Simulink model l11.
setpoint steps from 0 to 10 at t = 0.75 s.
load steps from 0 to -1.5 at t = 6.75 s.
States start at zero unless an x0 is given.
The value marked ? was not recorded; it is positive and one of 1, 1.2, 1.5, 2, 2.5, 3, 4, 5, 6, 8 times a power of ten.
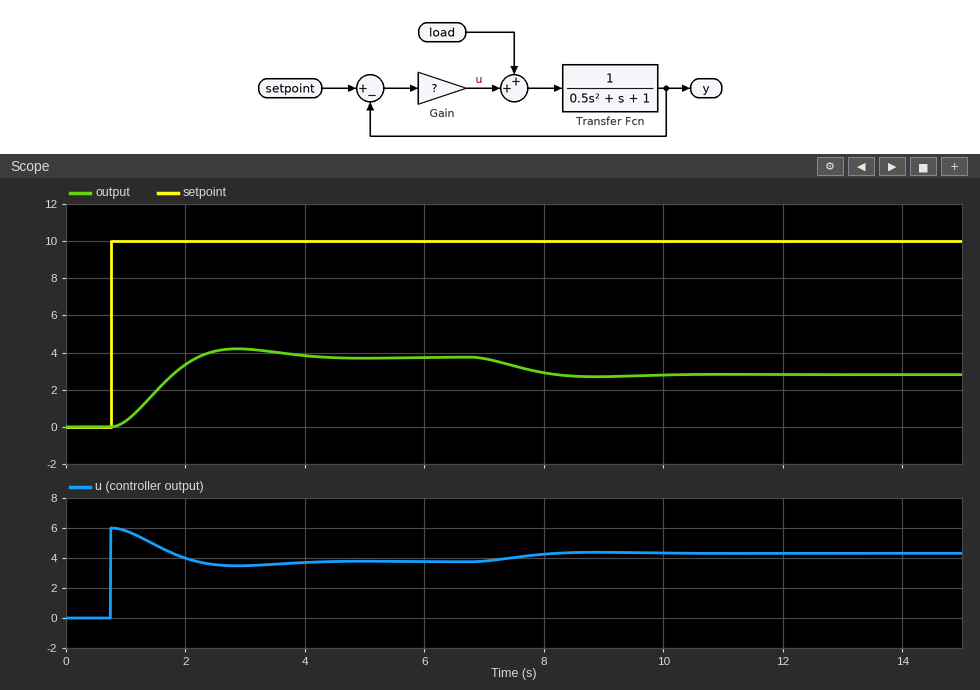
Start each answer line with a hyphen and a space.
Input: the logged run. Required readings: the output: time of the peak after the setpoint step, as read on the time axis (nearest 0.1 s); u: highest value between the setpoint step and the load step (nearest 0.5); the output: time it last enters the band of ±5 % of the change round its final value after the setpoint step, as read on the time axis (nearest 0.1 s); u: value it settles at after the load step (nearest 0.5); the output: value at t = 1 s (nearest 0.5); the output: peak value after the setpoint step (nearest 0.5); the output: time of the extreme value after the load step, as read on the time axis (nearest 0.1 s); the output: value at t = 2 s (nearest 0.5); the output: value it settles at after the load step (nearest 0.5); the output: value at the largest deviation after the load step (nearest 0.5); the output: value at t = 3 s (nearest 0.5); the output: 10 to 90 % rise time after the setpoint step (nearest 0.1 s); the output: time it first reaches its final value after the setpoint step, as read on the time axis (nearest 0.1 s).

- 2.9 s
- 6.0
- 3.7 s
- 4.5
- 0.5
- 4.0
- 8.9 s
- 3.5
- 3.0
- 2.5
- 4.0
- 1.0 s
- 2.2 s
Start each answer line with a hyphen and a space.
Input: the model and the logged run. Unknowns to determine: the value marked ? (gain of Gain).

- 0.6
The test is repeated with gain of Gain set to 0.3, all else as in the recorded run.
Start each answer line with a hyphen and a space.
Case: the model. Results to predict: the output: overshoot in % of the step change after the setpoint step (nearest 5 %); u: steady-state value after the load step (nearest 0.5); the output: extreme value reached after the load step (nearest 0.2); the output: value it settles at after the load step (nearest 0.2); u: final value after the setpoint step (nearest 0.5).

- 10 %
- 2.5
- 1.0
- 1.2
- 2.5
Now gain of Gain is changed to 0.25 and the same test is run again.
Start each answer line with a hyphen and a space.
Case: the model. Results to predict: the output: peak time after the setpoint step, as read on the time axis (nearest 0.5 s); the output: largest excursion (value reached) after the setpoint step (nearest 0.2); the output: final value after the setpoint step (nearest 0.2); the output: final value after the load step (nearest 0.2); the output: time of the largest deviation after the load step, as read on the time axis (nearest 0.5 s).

- 3.5 s
- 2.2
- 2.0
- 0.8
- 9.5 s
